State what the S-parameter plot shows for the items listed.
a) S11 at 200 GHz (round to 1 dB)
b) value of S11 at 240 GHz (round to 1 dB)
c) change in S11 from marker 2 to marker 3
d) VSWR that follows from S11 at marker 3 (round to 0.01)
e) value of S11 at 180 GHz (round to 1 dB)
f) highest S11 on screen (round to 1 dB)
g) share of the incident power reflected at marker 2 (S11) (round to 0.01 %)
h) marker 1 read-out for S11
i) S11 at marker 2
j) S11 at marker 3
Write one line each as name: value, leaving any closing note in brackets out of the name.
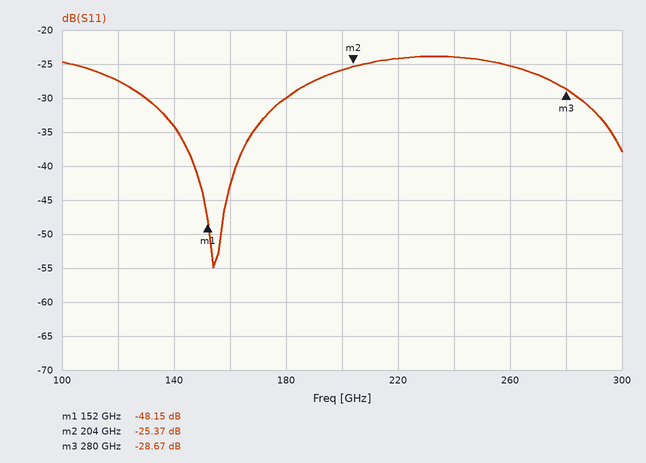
S11 at 200 GHz: -26 dB
value of S11 at 240 GHz: -24 dB
change in S11 from marker 2 to marker 3: -3.30 dB
VSWR that follows from S11 at marker 3: 1.08
value of S11 at 180 GHz: -30 dB
highest S11 on screen: -24 dB
share of the incident power reflected at marker 2 (S11): 0.29 %
marker 1 read-out for S11: -48.15 dB
S11 at marker 2: -25.37 dB
S11 at marker 3: -28.67 dB
